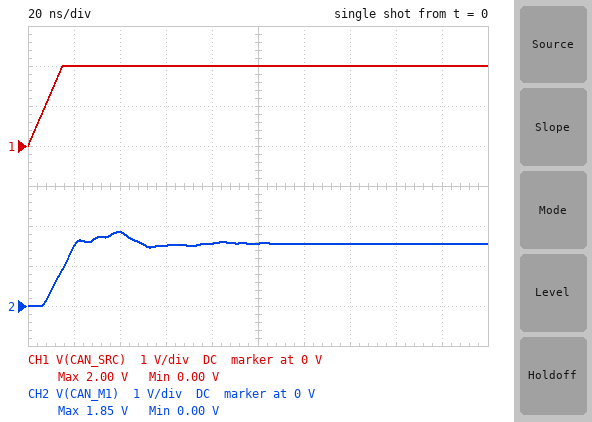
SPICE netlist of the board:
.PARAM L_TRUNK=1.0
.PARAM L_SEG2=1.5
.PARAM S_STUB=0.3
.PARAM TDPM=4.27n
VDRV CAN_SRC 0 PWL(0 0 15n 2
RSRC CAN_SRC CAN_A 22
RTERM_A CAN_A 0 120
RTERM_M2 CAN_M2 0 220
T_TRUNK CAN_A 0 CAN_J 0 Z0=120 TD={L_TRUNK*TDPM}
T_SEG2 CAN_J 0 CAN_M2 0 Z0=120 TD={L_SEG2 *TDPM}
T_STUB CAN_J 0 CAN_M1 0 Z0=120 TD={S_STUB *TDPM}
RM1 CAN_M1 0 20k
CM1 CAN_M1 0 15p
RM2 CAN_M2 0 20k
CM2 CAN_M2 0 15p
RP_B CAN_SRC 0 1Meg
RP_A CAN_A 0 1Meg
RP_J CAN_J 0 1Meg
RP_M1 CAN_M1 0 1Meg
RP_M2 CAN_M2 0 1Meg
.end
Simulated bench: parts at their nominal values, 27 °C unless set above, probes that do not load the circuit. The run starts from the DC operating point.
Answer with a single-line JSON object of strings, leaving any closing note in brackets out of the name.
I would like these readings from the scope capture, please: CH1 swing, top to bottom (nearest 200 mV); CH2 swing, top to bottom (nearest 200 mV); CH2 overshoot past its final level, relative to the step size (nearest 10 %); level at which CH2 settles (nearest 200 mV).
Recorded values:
{"CH1 swing, top to bottom": "2.0 V", "CH2 swing, top to bottom": "1.8 V", "CH2 overshoot past its final level, relative to the step size": "20 %", "level at which CH2 settles": "1.6 V"}
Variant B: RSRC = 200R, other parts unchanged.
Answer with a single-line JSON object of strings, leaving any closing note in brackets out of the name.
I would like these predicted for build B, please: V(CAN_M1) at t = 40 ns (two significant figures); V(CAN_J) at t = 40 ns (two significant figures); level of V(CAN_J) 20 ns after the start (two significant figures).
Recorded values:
{"V(CAN_M1) at t = 40 ns": "590 mV", "V(CAN_J) at t = 40 ns": "580 mV", "level of V(CAN_J) 20 ns after the start": "430 mV"}
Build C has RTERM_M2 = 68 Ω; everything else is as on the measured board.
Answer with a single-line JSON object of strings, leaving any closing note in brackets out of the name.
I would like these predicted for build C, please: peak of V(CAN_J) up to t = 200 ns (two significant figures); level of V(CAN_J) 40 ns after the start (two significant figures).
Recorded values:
{"peak of V(CAN_J) up to t = 200 ns": "1.5 V", "level of V(CAN_J) 40 ns after the start": "1.2 V"}
